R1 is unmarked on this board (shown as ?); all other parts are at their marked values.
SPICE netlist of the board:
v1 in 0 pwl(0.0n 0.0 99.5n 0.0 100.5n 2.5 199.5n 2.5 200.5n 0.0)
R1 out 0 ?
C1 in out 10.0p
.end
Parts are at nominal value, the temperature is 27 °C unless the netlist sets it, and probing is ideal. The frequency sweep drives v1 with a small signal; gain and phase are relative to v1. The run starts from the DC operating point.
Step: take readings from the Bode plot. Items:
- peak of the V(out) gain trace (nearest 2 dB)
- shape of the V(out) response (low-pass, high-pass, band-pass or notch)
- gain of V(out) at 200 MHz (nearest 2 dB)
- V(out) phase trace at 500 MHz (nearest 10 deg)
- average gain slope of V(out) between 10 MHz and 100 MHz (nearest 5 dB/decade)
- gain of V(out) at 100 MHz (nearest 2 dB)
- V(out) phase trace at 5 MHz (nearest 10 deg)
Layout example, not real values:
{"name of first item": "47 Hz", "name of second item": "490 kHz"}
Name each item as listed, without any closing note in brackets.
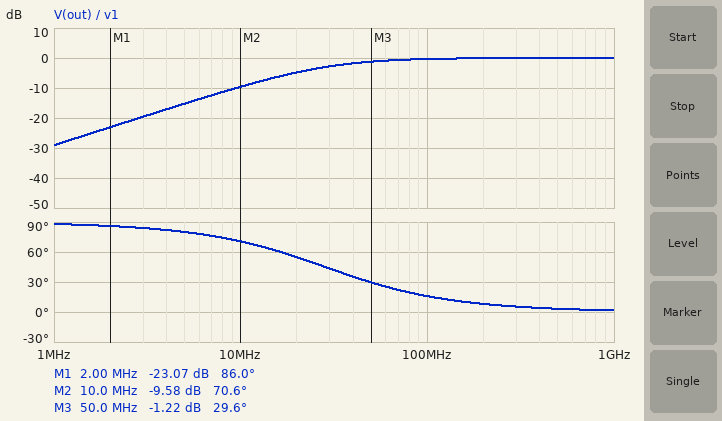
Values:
{"peak of the V(out) gain trace": "0 dB", "shape of the V(out) response": "high-pass", "gain of V(out) at 200 MHz": "0 dB", "V(out) phase trace at 500 MHz": "0 deg", "average gain slope of V(out) between 10 MHz and 100 MHz": "10 dB/decade", "gain of V(out) at 100 MHz": "0 dB", "V(out) phase trace at 5 MHz": "80 deg"}
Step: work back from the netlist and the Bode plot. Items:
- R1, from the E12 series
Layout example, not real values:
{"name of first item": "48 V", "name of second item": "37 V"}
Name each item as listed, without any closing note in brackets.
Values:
{"R1, from the E12 series": "560 Ω"}
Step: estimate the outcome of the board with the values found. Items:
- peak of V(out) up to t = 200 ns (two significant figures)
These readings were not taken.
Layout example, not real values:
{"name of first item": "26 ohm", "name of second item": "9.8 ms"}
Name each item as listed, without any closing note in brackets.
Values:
{"peak of V(out) up to t = 200 ns": "2.3 V"}
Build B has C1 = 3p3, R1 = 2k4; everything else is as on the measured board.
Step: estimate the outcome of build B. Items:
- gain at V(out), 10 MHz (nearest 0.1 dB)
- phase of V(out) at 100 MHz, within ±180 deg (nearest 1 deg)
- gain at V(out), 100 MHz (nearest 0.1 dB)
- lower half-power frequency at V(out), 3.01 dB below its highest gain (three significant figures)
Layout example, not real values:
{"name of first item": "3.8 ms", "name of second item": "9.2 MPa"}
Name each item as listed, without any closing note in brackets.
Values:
{"gain at V(out), 10 MHz": "-7.0 dB", "phase of V(out) at 100 MHz, within ±180 deg": "11 deg", "gain at V(out), 100 MHz": "-0.2 dB", "lower half-power frequency at V(out), 3.01 dB below its highest gain": "20.1 MHz"}
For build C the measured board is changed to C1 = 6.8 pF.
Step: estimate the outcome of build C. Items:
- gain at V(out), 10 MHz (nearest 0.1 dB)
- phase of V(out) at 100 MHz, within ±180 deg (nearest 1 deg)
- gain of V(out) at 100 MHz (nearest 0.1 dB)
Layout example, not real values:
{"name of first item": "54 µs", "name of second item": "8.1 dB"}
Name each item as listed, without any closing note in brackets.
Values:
{"gain at V(out), 10 MHz": "-12.7 dB", "phase of V(out) at 100 MHz, within ±180 deg": "23 deg", "gain of V(out) at 100 MHz": "-0.7 dB"}
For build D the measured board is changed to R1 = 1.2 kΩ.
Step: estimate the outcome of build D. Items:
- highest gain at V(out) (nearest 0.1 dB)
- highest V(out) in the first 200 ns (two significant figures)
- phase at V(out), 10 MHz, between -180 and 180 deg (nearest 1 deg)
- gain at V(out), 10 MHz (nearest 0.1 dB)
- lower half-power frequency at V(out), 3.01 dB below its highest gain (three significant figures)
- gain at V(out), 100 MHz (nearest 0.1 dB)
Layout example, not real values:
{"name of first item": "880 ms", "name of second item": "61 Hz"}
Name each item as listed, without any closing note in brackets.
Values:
{"highest gain at V(out)": "0 dB", "highest V(out) in the first 200 ns": "2.4 V", "phase at V(out), 10 MHz, between -180 and 180 deg": "53 deg", "gain at V(out), 10 MHz": "-4.4 dB", "lower half-power frequency at V(out), 3.01 dB below its highest gain": "13.3 MHz", "gain at V(out), 100 MHz": "-0.1 dB"}
